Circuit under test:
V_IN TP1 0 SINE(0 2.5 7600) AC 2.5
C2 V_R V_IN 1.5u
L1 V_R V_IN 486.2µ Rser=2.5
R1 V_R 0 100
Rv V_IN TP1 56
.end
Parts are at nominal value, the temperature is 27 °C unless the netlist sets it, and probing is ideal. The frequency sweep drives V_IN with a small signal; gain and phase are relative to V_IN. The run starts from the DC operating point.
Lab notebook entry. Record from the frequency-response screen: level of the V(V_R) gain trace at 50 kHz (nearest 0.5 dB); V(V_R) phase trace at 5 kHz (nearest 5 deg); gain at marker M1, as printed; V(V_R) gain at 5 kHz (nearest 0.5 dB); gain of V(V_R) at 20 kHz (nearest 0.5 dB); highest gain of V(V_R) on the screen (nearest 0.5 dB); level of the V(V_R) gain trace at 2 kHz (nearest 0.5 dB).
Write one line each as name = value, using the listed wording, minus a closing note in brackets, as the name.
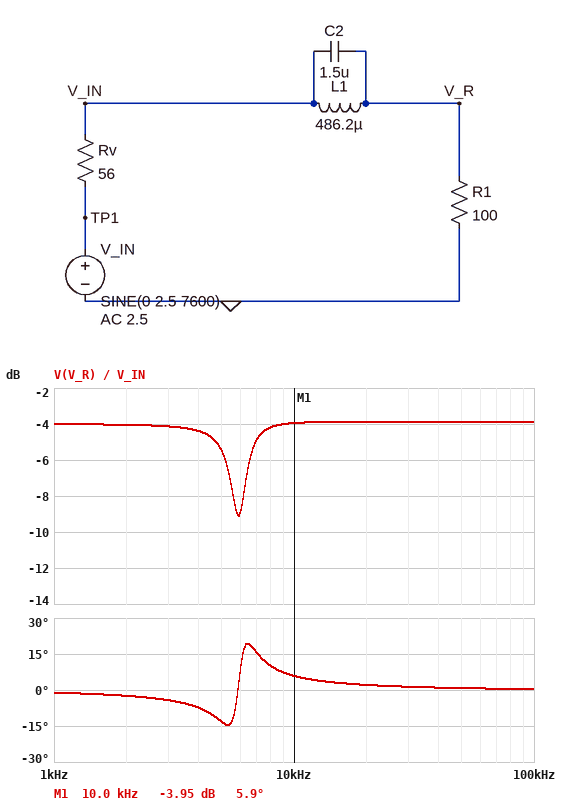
level of the V(V_R) gain trace at 50 kHz = -4.0 dB
V(V_R) phase trace at 5 kHz = -15 deg
gain at marker M1, as printed = -3.95 dB
V(V_R) gain at 5 kHz = -5.5 dB
gain of V(V_R) at 20 kHz = -4.0 dB
highest gain of V(V_R) on the screen = -4.0 dB
level of the V(V_R) gain trace at 2 kHz = -4.0 dB
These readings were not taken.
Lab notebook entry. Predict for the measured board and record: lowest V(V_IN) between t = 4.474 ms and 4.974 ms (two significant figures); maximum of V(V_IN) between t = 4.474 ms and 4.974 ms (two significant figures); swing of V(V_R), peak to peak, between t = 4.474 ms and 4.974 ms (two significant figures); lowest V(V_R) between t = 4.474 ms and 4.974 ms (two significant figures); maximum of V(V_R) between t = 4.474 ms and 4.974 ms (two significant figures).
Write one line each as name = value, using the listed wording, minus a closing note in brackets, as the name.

lowest V(V_IN) between t = 4.474 ms and 4.974 ms = -1.7 V
maximum of V(V_IN) between t = 4.474 ms and 4.974 ms = 1.7 V
swing of V(V_R), peak to peak, between t = 4.474 ms and 4.974 ms = 3.0 V
lowest V(V_R) between t = 4.474 ms and 4.974 ms = -1.5 V
maximum of V(V_R) between t = 4.474 ms and 4.974 ms = 1.5 V
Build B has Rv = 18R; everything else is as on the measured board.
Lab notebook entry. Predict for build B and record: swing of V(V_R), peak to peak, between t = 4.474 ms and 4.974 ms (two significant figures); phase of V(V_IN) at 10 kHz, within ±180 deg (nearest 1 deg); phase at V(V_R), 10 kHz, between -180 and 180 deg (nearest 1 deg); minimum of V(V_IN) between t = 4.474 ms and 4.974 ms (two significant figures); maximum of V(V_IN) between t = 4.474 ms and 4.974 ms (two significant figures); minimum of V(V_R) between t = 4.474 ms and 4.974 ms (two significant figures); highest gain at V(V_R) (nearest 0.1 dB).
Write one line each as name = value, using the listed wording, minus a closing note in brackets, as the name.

swing of V(V_R), peak to peak, between t = 4.474 ms and 4.974 ms = 3.9 V
phase of V(V_IN) at 10 kHz, within ±180 deg = -1 deg
phase at V(V_R), 10 kHz, between -180 and 180 deg = 8 deg
minimum of V(V_IN) between t = 4.474 ms and 4.974 ms = -2.2 V
maximum of V(V_IN) between t = 4.474 ms and 4.974 ms = 2.2 V
minimum of V(V_R) between t = 4.474 ms and 4.974 ms = -2.0 V
highest gain at V(V_R) = -1.4 dB
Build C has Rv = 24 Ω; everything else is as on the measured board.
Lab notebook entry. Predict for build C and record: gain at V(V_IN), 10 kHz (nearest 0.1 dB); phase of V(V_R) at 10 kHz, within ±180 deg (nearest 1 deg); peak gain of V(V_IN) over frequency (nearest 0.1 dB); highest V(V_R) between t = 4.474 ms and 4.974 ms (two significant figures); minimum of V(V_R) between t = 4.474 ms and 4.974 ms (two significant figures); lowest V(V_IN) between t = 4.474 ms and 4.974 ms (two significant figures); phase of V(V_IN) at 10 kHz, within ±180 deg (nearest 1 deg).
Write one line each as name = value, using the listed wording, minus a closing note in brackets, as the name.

gain at V(V_IN), 10 kHz = -1.8 dB
phase of V(V_R) at 10 kHz, within ±180 deg = 7 deg
peak gain of V(V_IN) over frequency = -0.9 dB
highest V(V_R) between t = 4.474 ms and 4.974 ms = 1.9 V
minimum of V(V_R) between t = 4.474 ms and 4.974 ms = -1.9 V
lowest V(V_IN) between t = 4.474 ms and 4.974 ms = -2.1 V
phase of V(V_IN) at 10 kHz, within ±180 deg = -2 deg
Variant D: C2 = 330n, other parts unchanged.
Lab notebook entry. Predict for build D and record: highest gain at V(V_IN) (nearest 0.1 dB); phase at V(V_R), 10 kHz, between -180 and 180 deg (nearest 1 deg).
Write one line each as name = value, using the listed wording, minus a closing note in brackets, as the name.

highest gain at V(V_IN) = -0.7 dB
phase at V(V_R), 10 kHz, between -180 and 180 deg = -25 deg
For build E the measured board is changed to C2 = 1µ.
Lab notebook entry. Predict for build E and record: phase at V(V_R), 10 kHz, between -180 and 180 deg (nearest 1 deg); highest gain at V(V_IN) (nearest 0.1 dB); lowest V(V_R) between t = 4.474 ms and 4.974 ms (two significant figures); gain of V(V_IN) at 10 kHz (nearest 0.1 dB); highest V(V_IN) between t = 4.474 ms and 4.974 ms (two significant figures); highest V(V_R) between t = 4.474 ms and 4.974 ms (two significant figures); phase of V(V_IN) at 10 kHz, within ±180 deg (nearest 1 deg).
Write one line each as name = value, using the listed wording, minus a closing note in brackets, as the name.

phase at V(V_R), 10 kHz, between -180 and 180 deg = 12 deg
highest gain at V(V_IN) = -1.5 dB
lowest V(V_R) between t = 4.474 ms and 4.974 ms = -910 mV
gain of V(V_IN) at 10 kHz = -3.5 dB
highest V(V_IN) between t = 4.474 ms and 4.974 ms = 2.0 V
highest V(V_R) between t = 4.474 ms and 4.974 ms = 910 mV
phase of V(V_IN) at 10 kHz, within ±180 deg = -6 deg
